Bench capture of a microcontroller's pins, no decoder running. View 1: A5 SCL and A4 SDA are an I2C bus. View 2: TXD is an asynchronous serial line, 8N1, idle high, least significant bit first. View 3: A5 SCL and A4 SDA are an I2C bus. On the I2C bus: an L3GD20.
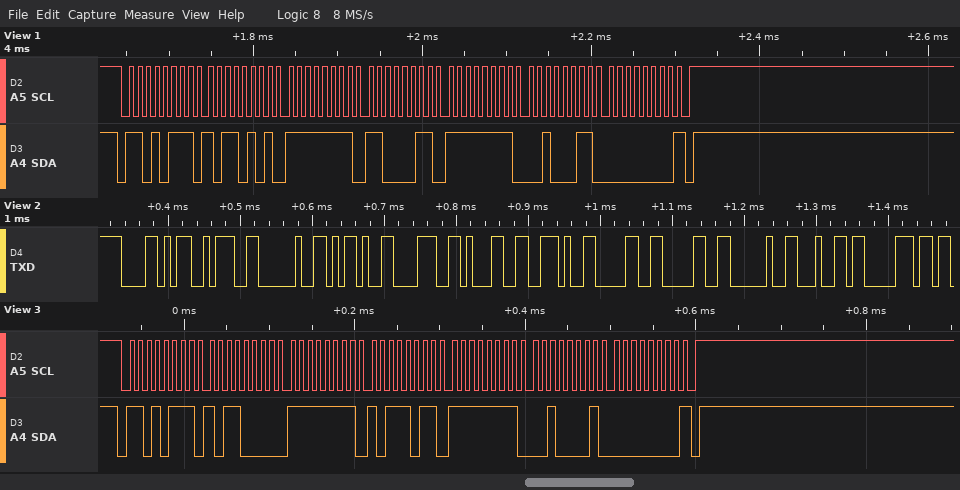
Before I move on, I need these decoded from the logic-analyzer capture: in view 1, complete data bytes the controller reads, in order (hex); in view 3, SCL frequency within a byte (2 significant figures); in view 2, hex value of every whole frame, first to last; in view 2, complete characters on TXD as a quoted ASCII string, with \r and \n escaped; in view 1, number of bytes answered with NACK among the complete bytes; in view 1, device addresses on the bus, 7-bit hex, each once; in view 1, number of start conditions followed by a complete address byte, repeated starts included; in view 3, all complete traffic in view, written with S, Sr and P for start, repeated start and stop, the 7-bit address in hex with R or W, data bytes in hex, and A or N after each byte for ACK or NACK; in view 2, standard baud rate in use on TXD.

B5 FF C3 FF 23 00
100 kHz
58 3A 20 2D 38 31 2E 30 30 20 64 70
"X: -81.00 dp"
1
0x6B
1
S 6BR A B0 A FF A BB A FF A 21 A 00 N P
115200 baud
